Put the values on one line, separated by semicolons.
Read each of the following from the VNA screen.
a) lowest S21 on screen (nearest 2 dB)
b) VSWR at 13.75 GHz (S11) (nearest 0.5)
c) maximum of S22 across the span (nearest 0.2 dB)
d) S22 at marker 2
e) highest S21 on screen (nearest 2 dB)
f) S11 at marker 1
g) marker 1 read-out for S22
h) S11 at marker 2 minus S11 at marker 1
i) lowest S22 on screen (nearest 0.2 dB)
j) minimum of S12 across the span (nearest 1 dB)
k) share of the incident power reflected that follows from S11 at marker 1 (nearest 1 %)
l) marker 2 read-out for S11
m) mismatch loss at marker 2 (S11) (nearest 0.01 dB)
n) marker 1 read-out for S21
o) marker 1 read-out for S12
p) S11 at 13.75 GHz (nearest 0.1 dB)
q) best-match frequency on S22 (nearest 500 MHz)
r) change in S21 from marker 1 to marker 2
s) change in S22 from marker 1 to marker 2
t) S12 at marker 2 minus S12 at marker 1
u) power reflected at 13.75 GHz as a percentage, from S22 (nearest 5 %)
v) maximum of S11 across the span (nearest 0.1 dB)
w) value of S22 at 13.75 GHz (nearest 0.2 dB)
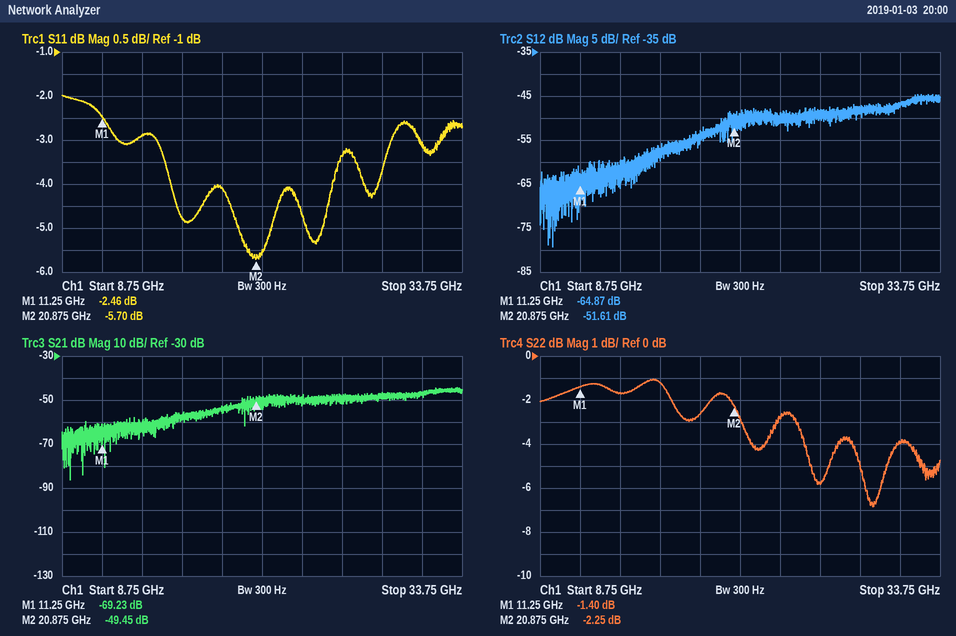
-86 dB; 6.0; -1.0 dB; -2.25 dB; -44 dB; -2.46 dB; -1.40 dB; -3.24 dB; -6.8 dB; -79 dB; 57 %; -5.70 dB; 1.36 dB; -69.23 dB; -64.87 dB; -2.9 dB; 29.5 GHz; 19.78 dB; -0.85 dB; 13.26 dB; 70 %; -2.0 dB; -1.6 dB
